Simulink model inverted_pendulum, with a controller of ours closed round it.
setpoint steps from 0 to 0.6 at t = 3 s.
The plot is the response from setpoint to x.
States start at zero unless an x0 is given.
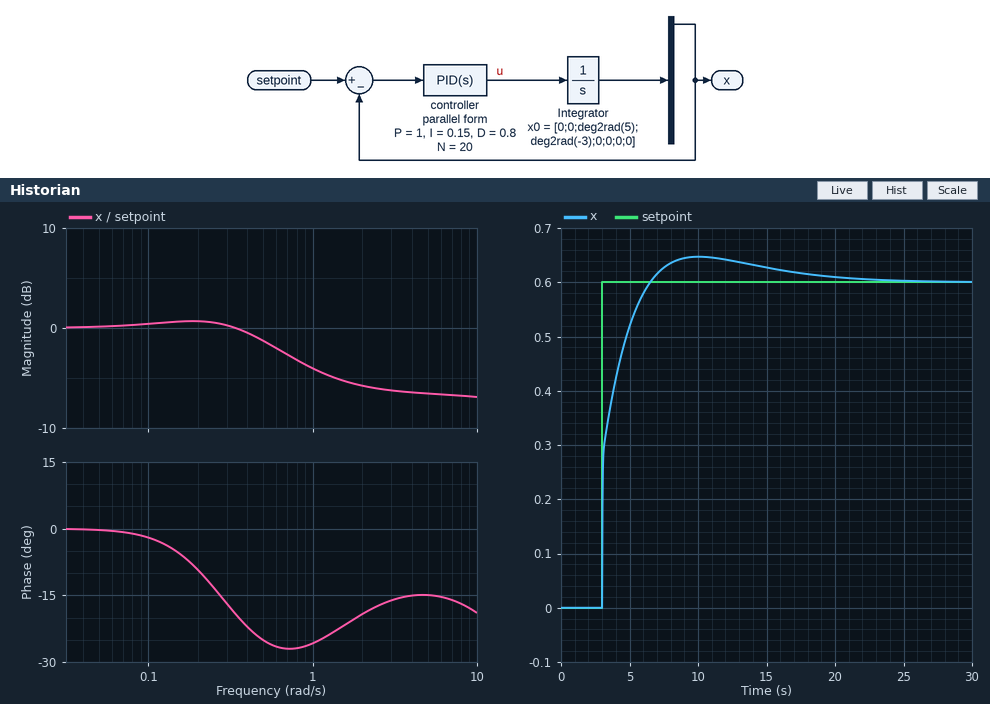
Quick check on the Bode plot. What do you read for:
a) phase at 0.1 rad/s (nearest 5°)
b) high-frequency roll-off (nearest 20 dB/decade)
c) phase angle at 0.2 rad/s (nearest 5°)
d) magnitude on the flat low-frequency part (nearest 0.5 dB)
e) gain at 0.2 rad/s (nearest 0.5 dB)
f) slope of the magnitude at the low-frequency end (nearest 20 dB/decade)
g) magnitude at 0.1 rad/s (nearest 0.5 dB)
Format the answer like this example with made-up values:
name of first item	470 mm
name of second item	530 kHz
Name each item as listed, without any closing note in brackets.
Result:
phase at 0.1 rad/s	0°
high-frequency roll-off	0 dB/decade
phase angle at 0.2 rad/s	-10°
magnitude on the flat low-frequency part	0.0 dB
gain at 0.2 rad/s	0.5 dB
slope of the magnitude at the low-frequency end	0 dB/decade
magnitude at 0.1 rad/s	0.5 dB
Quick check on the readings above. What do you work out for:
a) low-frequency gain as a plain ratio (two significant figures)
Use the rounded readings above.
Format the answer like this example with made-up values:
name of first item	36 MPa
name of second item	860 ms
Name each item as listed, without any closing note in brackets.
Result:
low-frequency gain as a plain ratio	1.0
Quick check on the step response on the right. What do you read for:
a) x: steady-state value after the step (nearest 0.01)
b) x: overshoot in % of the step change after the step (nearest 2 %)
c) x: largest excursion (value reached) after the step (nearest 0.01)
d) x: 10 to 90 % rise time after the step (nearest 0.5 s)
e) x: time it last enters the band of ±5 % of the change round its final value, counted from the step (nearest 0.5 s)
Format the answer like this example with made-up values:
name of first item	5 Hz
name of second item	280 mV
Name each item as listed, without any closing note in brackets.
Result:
x: steady-state value after the step	0.60
x: overshoot in % of the step change after the step	8 %
x: largest excursion (value reached) after the step	0.65
x: 10 to 90 % rise time after the step	2.5 s
x: time it last enters the band of ±5 % of the change round its final value, counted from the step	11.5 s
